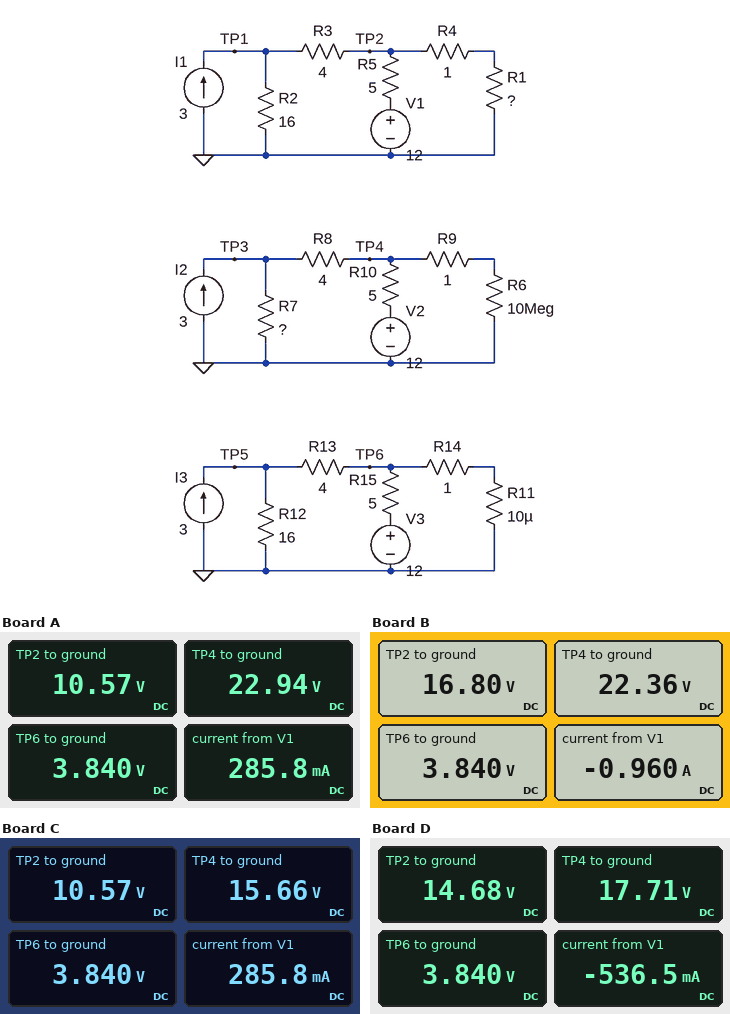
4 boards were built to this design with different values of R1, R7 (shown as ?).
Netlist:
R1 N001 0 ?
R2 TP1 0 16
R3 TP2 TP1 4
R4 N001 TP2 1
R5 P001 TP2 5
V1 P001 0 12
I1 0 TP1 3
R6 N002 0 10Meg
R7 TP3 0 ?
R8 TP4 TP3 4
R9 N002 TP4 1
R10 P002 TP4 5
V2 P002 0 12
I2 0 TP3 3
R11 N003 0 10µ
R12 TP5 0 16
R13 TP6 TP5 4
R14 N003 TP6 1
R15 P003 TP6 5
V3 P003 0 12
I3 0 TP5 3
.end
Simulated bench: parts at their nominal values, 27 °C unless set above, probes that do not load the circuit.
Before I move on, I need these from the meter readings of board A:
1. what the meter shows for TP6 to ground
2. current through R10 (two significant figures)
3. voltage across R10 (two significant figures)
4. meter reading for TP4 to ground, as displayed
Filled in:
3.840 V
2.2 A
11 V
22.94 V
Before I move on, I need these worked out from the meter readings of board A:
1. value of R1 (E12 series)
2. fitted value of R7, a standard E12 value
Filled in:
3.9 Ω
39 Ω
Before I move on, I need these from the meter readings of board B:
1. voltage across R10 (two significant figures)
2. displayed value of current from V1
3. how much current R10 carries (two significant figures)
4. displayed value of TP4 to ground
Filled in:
10 V
-0.960 A
2.1 A
22.36 V
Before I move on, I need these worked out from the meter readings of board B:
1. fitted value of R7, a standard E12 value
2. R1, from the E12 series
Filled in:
33 Ω
27 Ω
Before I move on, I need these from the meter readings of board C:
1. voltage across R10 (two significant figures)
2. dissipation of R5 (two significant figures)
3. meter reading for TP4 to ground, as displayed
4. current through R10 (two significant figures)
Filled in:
3.7 V
410 mW
15.66 V
730 mA
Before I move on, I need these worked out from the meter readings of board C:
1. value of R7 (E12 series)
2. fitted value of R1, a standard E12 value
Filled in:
8.2 Ω
3.9 Ω
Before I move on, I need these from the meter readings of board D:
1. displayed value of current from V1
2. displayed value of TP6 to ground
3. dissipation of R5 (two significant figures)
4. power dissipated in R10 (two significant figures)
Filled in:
-536.5 mA
3.840 V
1.4 W
6.5 W
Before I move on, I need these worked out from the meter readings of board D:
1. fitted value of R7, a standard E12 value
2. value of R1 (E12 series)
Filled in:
12 Ω
12 Ω
